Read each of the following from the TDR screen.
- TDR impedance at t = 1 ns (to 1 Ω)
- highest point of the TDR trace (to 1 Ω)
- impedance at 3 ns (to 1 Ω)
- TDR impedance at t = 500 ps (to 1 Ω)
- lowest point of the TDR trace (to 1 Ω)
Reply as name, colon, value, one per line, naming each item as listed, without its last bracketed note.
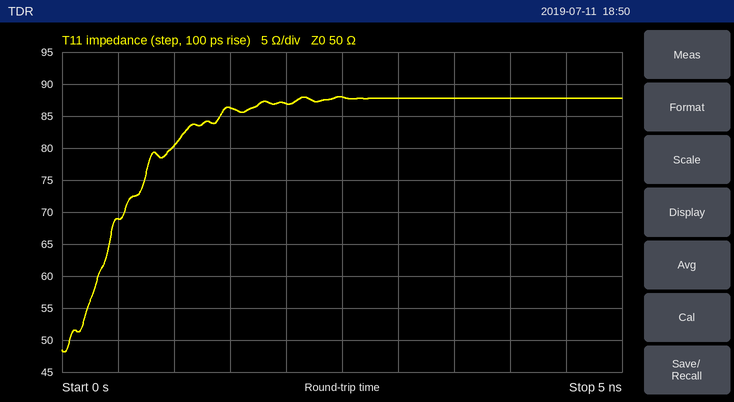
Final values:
TDR impedance at t = 1 ns: 80 Ω
highest point of the TDR trace: 88 Ω
impedance at 3 ns: 88 Ω
TDR impedance at t = 500 ps: 69 Ω
lowest point of the TDR trace: 48 Ω
